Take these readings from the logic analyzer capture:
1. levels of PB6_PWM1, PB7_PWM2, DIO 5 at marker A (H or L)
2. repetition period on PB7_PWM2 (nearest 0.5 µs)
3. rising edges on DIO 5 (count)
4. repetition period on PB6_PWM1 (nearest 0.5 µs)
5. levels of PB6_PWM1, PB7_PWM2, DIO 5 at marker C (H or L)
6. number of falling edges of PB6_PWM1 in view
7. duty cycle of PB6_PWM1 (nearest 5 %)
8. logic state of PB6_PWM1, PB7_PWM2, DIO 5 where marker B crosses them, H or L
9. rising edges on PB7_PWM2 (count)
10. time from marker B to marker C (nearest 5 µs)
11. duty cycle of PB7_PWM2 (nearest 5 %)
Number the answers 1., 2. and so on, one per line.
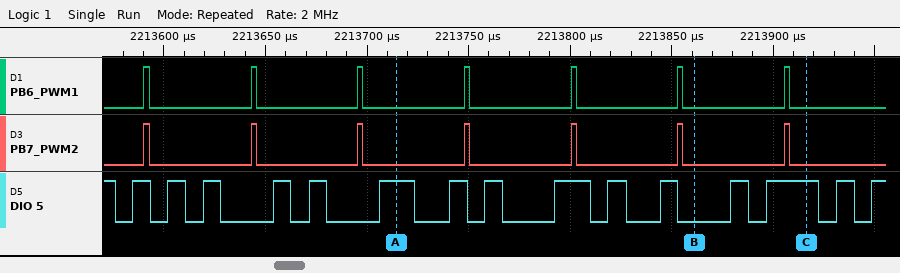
1. PB6_PWM1=L, PB7_PWM2=L, DIO 5=H
2. 52.5 µs
3. 15
4. 52.5 µs
5. PB6_PWM1=L, PB7_PWM2=L, DIO 5=H
6. 7
7. 5 %
8. PB6_PWM1=L, PB7_PWM2=L, DIO 5=L
9. 7
10. 55 µs
11. 5 %
